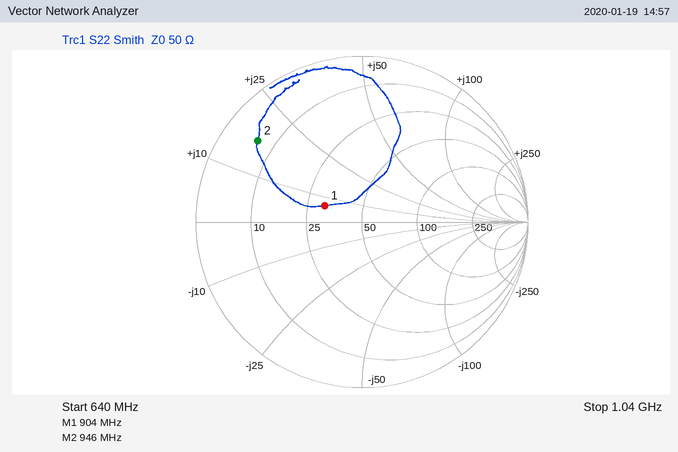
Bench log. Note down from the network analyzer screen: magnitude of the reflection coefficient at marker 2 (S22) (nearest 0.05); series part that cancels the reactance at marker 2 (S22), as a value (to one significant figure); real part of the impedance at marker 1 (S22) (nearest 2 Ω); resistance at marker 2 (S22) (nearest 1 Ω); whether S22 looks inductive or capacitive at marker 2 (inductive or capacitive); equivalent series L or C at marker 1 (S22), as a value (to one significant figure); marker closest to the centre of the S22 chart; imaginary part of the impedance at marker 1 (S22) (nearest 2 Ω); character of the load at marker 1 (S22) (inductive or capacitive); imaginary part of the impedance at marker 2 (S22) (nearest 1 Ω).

0.80
10 pF
32 Ω
6 Ω
inductive
1 nH
marker 1
+6 Ω
inductive
+17 Ω
